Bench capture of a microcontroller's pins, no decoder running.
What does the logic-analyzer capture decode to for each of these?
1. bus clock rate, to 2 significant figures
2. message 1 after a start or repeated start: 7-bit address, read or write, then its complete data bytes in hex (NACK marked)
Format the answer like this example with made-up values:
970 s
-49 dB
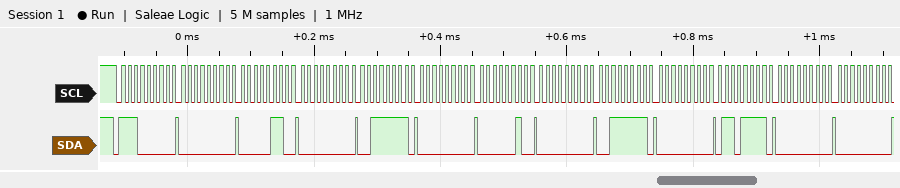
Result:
100 kHz
0x70 write: 00 06 00 3F 00 02 00 3F 00 6F 00 00
